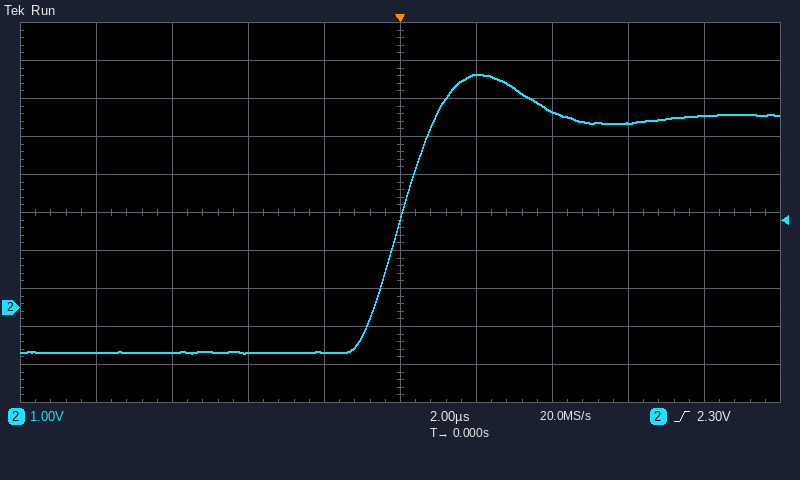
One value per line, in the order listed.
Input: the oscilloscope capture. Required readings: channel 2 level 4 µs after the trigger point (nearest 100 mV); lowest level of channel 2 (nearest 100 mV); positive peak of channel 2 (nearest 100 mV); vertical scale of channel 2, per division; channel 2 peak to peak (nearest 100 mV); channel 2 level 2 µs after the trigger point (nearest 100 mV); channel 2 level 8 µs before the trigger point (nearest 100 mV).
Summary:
5.2 V
-1.2 V
6.1 V
1 V
7.3 V
6.1 V
-1.2 V
